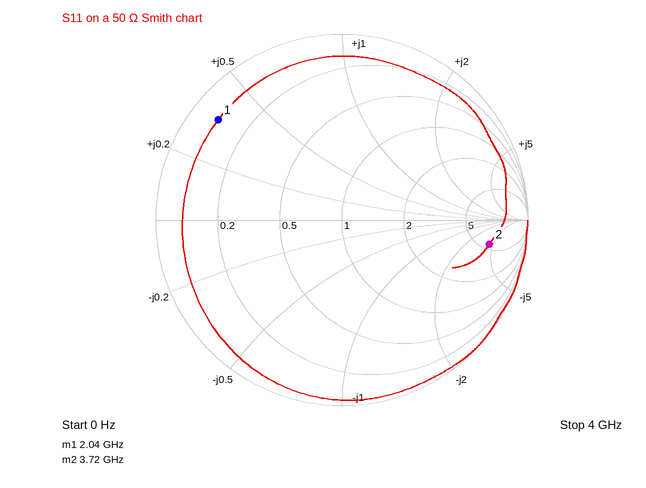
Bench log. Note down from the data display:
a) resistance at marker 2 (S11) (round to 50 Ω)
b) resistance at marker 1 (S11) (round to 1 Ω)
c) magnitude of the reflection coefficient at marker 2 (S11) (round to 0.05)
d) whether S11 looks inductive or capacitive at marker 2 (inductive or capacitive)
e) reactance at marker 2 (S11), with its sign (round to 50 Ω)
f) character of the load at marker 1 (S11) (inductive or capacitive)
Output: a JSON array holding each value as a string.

["300 Ω", "4 Ω", "0.80", "capacitive", "-200 Ω", "inductive"]
